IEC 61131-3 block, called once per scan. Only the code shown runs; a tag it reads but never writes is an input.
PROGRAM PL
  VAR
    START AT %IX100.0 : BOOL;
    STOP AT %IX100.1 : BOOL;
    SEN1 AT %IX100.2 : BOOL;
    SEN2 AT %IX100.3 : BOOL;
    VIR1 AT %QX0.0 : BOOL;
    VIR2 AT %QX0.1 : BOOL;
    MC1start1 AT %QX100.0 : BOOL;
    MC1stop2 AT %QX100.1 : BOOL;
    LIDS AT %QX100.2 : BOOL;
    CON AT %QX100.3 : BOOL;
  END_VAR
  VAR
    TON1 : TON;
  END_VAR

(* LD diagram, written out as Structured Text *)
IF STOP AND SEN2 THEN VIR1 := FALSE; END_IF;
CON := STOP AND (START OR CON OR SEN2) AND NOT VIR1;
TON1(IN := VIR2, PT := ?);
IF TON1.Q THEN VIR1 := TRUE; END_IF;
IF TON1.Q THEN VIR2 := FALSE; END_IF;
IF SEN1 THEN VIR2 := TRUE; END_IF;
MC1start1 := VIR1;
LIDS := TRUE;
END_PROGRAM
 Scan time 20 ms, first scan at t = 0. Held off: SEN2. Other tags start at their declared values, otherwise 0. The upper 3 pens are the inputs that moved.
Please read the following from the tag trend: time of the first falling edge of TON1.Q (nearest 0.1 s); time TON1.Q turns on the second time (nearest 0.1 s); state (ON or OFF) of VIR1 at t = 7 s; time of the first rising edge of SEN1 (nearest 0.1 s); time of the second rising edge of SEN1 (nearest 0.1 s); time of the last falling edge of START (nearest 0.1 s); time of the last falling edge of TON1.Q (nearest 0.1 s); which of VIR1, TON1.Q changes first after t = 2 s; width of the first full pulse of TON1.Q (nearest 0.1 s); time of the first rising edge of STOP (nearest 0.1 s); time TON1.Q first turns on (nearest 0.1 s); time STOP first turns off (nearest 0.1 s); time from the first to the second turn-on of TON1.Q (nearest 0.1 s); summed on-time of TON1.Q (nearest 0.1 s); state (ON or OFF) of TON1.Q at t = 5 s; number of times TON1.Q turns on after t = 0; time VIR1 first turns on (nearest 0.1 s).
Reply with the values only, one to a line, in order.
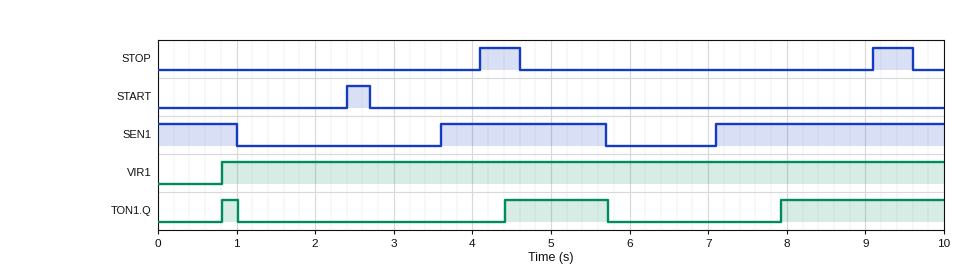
1.0 s
4.4 s
ON
3.6 s
7.1 s
2.7 s
5.7 s
TON1.Q
0.2 s
4.1 s
0.8 s
4.6 s
3.6 s
3.6 s
ON
3
0.8 s
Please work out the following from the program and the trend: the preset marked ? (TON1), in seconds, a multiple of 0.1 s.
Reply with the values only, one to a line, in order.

0.8 s
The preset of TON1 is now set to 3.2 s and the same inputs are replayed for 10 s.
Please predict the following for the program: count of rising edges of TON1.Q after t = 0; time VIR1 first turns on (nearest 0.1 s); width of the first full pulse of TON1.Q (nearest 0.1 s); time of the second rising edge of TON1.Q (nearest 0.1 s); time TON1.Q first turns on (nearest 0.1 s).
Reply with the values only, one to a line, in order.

2
3.2 s
0.0 s
6.8 s
3.2 s
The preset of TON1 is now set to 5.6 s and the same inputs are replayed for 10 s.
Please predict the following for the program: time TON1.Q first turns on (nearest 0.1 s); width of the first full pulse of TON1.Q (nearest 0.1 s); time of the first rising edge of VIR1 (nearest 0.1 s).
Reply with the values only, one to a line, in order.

5.6 s
0.1 s
5.6 s
